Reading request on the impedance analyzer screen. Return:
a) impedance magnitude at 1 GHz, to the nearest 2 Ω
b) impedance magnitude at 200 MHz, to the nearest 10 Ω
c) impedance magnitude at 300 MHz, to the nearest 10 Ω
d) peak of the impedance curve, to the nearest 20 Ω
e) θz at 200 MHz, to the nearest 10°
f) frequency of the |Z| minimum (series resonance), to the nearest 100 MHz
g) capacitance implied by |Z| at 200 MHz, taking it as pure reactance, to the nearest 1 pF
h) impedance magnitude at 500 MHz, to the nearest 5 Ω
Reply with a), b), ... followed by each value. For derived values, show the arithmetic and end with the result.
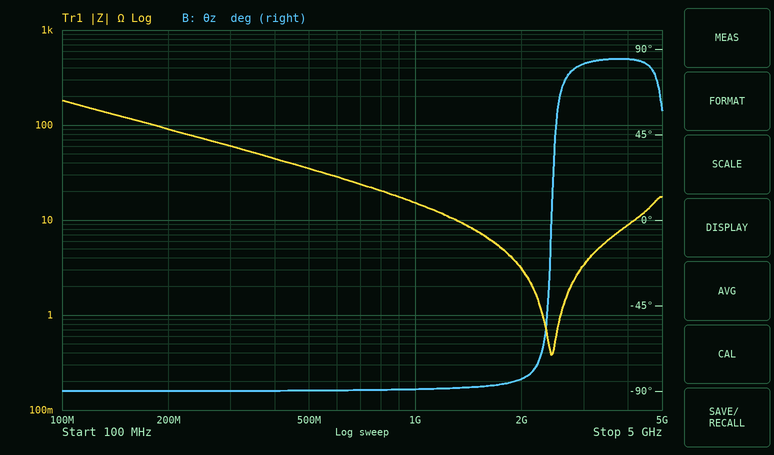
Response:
a) 16 Ω
b) 90 Ω
c) 60 Ω
d) 180 Ω
e) -90°
f) 2.4 GHz
g) C = 1/(2π × 200 MHz × 90 Ω) ≈ 9 pF
h) 35 Ω
